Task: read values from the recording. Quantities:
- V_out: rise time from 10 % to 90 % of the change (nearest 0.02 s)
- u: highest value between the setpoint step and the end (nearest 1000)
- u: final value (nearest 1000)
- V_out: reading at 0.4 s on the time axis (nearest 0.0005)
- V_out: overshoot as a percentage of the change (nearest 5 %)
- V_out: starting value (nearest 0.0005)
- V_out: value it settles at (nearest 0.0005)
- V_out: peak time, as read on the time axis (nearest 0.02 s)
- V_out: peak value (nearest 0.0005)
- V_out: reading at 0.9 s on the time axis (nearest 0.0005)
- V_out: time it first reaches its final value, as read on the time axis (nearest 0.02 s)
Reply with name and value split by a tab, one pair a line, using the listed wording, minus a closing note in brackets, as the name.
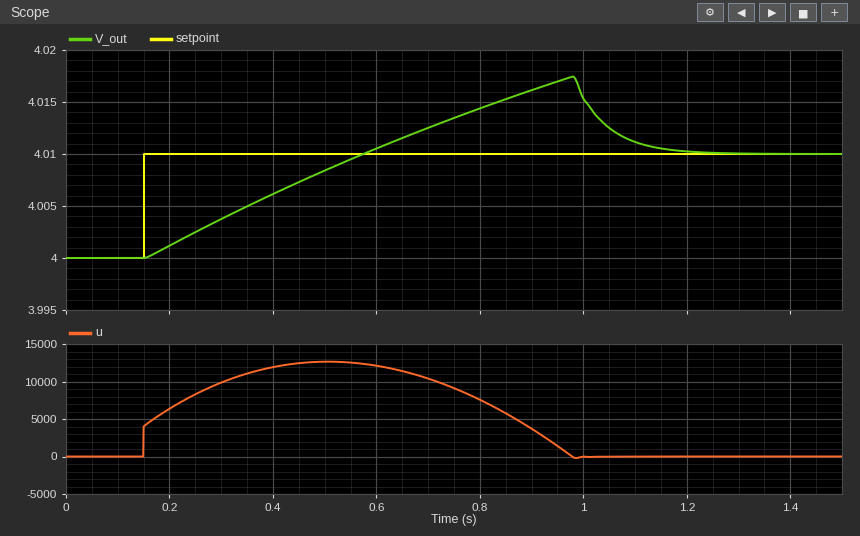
V_out: rise time from 10 % to 90 % of the change	0.34 s
u: highest value between the setpoint step and the end	13000
u: final value	0
V_out: reading at 0.4 s on the time axis	4.0060
V_out: overshoot as a percentage of the change	75 %
V_out: starting value	4.0000
V_out: value it settles at	4.0100
V_out: peak time, as read on the time axis	0.98 s
V_out: peak value	4.0175
V_out: reading at 0.9 s on the time axis	4.0160
V_out: time it first reaches its final value, as read on the time axis	0.58 s
